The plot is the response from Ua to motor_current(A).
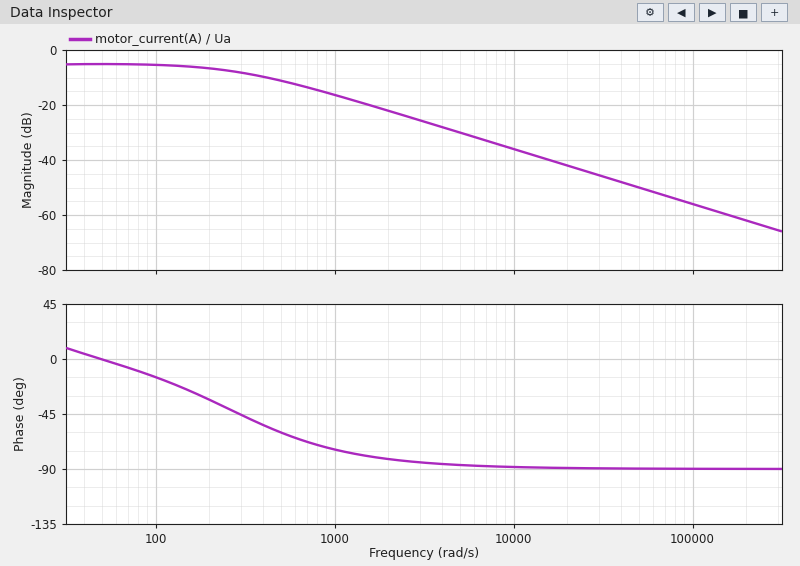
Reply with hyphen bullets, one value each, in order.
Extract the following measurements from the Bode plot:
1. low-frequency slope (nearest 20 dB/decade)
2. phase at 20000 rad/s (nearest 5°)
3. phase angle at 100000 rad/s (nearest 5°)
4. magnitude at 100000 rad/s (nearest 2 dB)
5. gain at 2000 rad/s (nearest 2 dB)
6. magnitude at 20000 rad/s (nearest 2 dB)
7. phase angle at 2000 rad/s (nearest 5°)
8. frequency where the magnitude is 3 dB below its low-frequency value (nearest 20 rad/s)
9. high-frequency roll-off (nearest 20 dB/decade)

- 0 dB/decade
- -90°
- -90°
- -56 dB
- -22 dB
- -42 dB
- -80°
- 300 rad/s
- -20 dB/decade
